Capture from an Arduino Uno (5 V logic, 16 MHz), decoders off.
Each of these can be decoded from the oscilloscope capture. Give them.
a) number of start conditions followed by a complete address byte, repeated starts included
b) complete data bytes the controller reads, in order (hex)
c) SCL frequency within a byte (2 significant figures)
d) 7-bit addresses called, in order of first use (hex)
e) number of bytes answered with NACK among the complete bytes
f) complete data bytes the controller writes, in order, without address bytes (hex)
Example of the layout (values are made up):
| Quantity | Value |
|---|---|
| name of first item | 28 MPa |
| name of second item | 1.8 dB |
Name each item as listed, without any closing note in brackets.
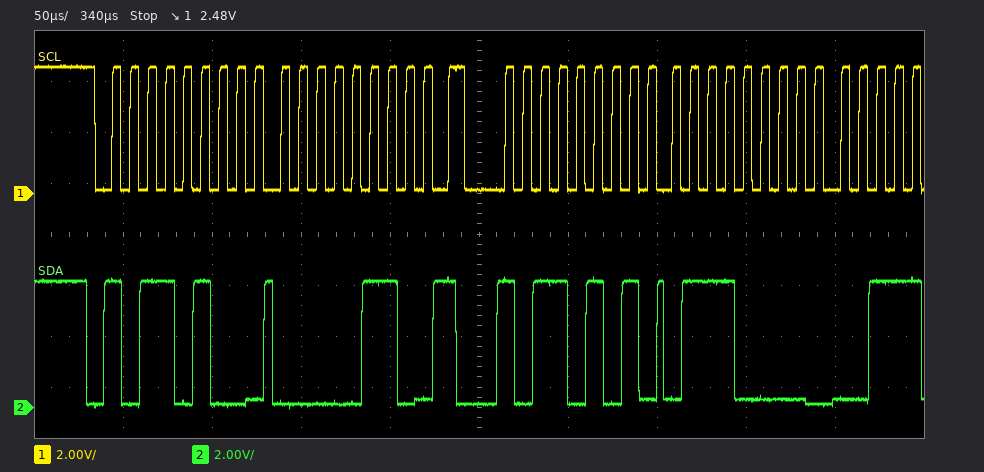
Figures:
| Quantity | Value |
|---|---|
| number of start conditions followed by a complete address byte, repeated starts included | 2 |
| complete data bytes the controller reads, in order | 70 |
| SCL frequency within a byte | 100 kHz |
| 7-bit addresses called, in order of first use | 0x5A |
| number of bytes answered with NACK among the complete bytes | 0 |
| complete data bytes the controller writes, in order, without address bytes | 06 |
